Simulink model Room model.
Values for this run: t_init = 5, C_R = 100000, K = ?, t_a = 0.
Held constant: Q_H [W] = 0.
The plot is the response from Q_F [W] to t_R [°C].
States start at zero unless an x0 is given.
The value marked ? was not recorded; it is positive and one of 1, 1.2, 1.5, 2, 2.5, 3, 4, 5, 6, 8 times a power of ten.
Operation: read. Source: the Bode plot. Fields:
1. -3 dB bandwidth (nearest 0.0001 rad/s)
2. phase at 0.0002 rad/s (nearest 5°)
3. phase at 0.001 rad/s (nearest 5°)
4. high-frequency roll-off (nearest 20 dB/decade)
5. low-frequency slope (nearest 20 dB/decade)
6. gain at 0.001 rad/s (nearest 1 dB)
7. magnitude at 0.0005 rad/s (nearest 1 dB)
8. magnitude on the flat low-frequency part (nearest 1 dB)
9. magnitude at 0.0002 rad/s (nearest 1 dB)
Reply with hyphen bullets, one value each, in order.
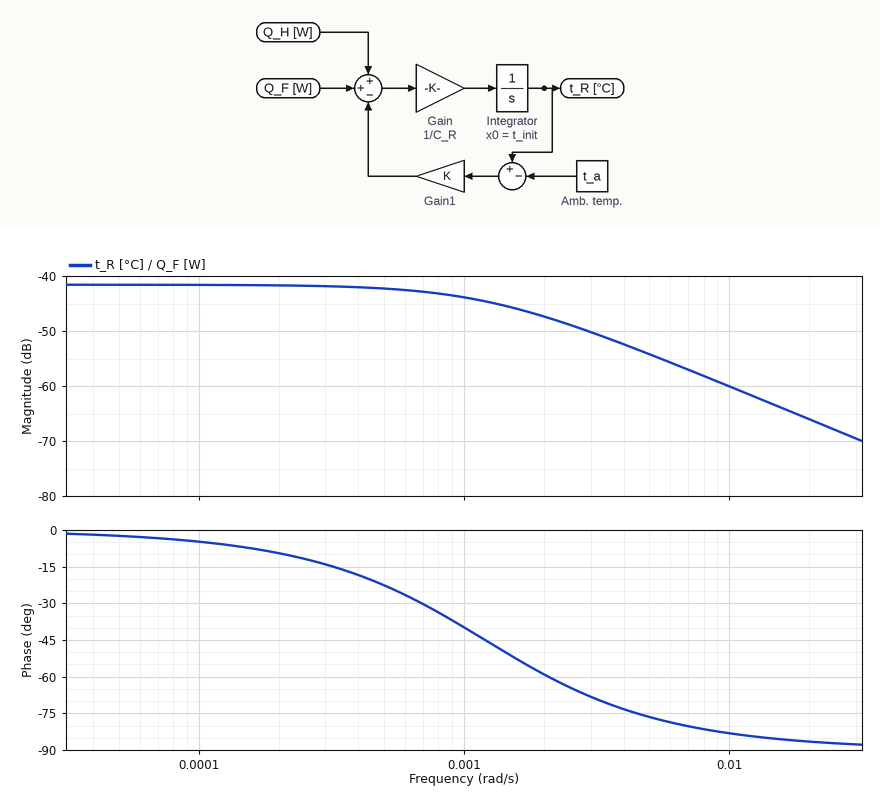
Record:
- 0.0012 rad/s
- -10°
- -40°
- -20 dB/decade
- 0 dB/decade
- -44 dB
- -42 dB
- -42 dB
- -42 dB
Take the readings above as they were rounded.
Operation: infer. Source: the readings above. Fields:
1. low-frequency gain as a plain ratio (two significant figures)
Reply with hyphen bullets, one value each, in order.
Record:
- 0.0079
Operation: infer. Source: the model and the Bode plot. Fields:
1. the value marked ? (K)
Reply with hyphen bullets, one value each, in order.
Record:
- 120
